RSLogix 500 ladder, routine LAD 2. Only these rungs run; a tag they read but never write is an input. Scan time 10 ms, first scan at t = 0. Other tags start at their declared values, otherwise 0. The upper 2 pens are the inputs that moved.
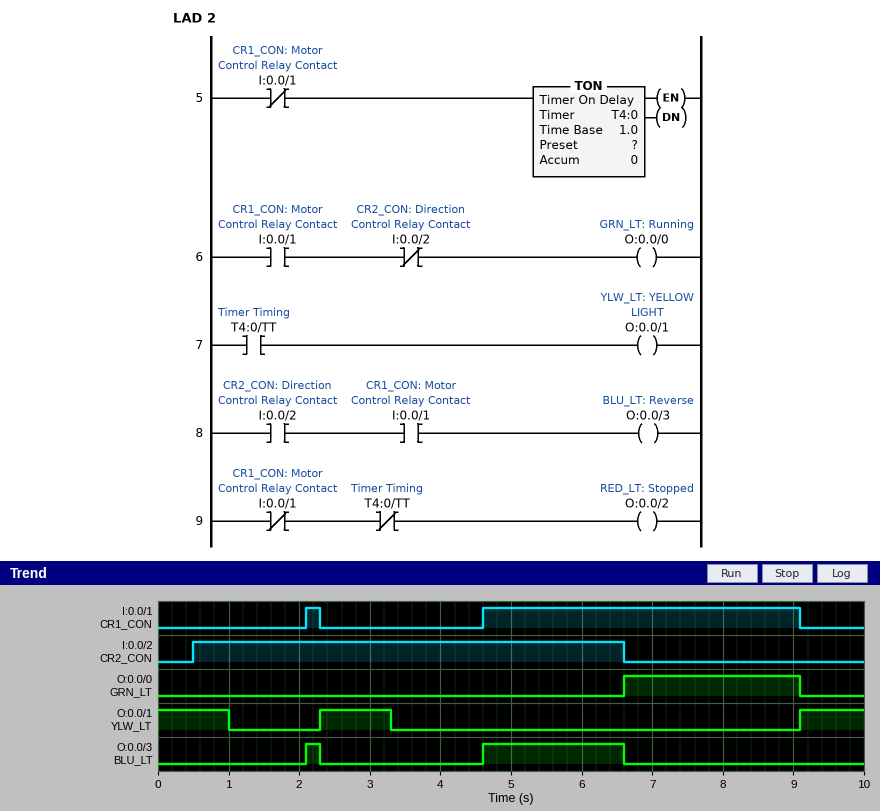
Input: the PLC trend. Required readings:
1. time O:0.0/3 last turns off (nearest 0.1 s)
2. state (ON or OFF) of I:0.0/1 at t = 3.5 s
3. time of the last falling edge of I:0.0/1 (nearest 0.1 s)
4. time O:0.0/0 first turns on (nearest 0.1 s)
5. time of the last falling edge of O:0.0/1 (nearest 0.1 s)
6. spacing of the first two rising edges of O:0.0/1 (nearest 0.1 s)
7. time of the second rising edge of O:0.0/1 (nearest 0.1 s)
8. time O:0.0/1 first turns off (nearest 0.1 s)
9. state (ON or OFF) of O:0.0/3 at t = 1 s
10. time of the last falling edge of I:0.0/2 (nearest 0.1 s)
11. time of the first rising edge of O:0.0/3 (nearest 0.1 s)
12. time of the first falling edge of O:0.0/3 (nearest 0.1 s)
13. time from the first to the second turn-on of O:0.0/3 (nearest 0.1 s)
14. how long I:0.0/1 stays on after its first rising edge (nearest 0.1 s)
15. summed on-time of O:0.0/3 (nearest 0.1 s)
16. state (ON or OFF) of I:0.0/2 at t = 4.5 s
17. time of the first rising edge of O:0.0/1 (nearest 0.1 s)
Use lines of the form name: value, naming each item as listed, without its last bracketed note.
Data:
time O:0.0/3 last turns off: 6.6 s
state (ON or OFF) of I:0.0/1 at t = 3.5 s: OFF
time of the last falling edge of I:0.0/1: 9.1 s
time O:0.0/0 first turns on: 6.6 s
time of the last falling edge of O:0.0/1: 3.3 s
spacing of the first two rising edges of O:0.0/1: 6.8 s
time of the second rising edge of O:0.0/1: 9.1 s
time O:0.0/1 first turns off: 1.0 s
state (ON or OFF) of O:0.0/3 at t = 1 s: OFF
time of the last falling edge of I:0.0/2: 6.6 s
time of the first rising edge of O:0.0/3: 2.1 s
time of the first falling edge of O:0.0/3: 2.3 s
time from the first to the second turn-on of O:0.0/3: 2.5 s
how long I:0.0/1 stays on after its first rising edge: 0.2 s
summed on-time of O:0.0/3: 2.2 s
state (ON or OFF) of I:0.0/2 at t = 4.5 s: ON
time of the first rising edge of O:0.0/1: 2.3 s
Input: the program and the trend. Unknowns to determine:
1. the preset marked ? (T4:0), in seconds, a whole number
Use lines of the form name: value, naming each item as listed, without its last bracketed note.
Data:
the preset marked ? (T4:0), in seconds, a whole number: 1 s
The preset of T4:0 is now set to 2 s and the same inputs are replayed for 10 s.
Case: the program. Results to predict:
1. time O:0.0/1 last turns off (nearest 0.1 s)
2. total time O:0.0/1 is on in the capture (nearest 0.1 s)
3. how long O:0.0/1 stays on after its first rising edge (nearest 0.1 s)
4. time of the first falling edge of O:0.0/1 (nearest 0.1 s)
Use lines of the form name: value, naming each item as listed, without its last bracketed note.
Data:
time O:0.0/1 last turns off: 4.3 s
total time O:0.0/1 is on in the capture: 4.9 s
how long O:0.0/1 stays on after its first rising edge: 2.0 s
time of the first falling edge of O:0.0/1: 2.0 s
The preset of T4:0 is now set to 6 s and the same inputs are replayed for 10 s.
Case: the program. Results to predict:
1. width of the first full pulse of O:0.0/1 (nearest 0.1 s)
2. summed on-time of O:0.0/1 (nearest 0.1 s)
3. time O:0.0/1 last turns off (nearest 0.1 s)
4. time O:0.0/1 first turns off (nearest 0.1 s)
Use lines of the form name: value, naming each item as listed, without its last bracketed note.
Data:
width of the first full pulse of O:0.0/1: 2.3 s
summed on-time of O:0.0/1: 5.3 s
time O:0.0/1 last turns off: 4.6 s
time O:0.0/1 first turns off: 2.1 s
